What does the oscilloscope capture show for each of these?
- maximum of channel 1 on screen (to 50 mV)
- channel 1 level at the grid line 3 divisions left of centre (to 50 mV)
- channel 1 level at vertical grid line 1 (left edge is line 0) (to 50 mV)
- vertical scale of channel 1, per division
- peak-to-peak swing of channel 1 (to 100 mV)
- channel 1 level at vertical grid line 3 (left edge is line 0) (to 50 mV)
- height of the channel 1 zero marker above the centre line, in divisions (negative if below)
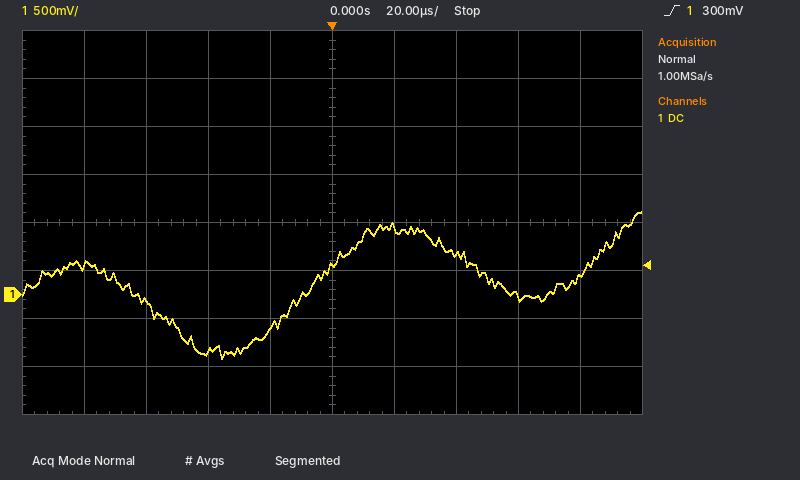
850 mV
-50 mV
300 mV
500 mV
1.50 V
-600 mV
-1.5 div
